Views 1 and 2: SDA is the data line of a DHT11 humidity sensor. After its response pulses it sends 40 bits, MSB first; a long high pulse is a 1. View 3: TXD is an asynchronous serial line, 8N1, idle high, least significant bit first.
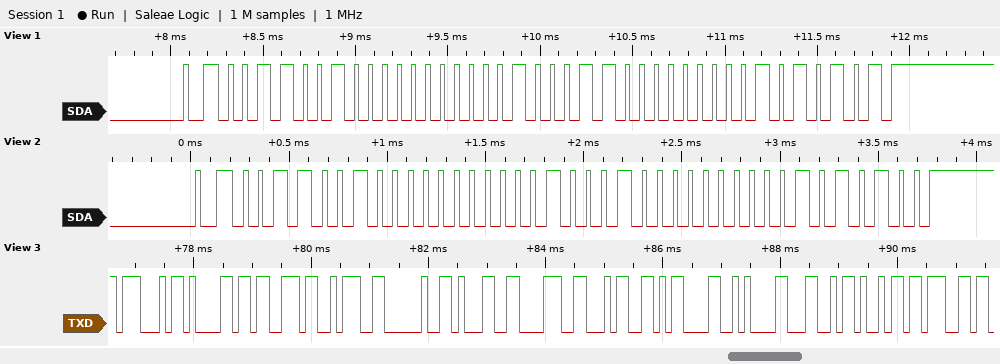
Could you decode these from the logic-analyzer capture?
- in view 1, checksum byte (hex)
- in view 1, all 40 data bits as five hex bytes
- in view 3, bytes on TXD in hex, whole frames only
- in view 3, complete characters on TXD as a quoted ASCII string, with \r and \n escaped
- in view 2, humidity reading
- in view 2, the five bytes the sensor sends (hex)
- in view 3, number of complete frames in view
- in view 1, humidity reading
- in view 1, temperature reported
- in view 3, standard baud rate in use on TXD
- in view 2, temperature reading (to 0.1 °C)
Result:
0x55
32 00 23 00 55
47 61 73 3A 20 31 38 34 0D 0A 4C 69 67
"Gas: 184\r\nLig"
50 %
32 00 22 00 54
13
50 %
35.0 °C
9600 baud
34.0 °C
